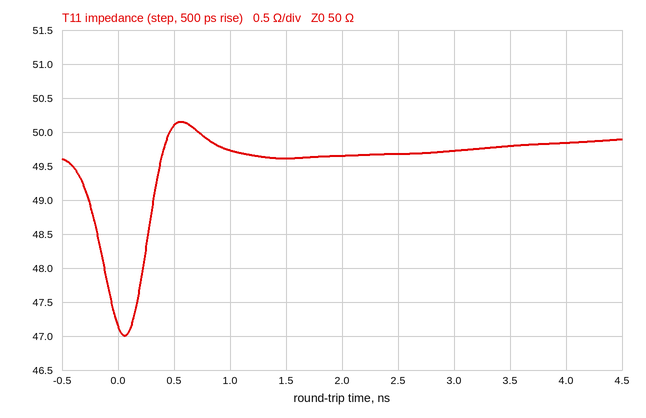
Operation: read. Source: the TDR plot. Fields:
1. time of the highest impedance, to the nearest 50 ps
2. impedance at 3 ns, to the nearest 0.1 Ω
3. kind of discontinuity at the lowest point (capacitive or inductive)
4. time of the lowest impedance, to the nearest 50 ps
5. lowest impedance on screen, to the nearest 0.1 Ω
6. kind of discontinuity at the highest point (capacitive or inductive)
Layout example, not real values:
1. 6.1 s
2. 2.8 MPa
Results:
1. 550 ps
2. 49.7 Ω
3. capacitive
4. 50 ps
5. 47.0 Ω
6. inductive
